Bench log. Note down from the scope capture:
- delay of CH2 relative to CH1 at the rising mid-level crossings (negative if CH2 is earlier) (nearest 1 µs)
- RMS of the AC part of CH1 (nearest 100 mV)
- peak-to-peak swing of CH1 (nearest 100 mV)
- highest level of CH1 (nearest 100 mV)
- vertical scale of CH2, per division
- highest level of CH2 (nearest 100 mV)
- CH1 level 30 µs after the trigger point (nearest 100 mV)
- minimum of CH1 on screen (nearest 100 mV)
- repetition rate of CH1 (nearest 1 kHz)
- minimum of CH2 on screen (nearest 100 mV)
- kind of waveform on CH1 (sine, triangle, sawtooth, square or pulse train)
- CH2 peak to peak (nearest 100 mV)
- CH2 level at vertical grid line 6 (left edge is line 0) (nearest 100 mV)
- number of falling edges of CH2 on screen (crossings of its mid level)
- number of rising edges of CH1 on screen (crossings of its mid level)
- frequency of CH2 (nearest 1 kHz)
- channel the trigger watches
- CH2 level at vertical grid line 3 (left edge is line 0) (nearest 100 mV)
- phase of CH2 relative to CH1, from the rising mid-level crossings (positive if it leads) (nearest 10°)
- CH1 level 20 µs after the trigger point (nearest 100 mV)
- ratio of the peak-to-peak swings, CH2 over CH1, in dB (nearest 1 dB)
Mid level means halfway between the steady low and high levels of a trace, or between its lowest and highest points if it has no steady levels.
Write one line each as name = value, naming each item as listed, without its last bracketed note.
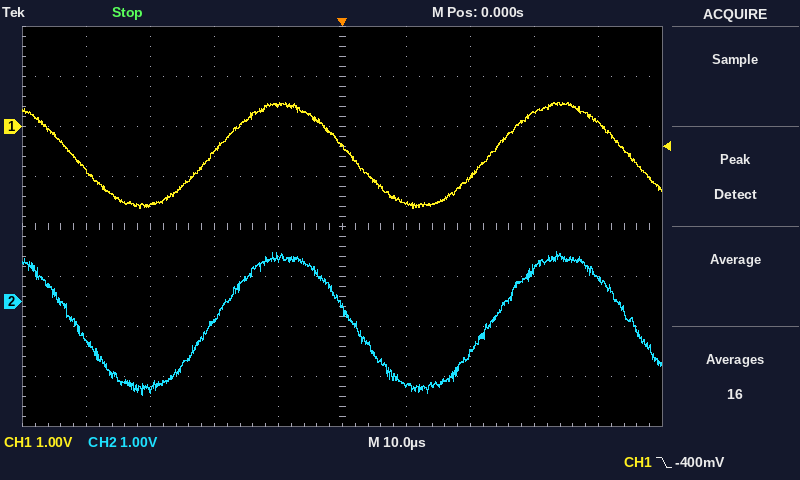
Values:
delay of CH2 relative to CH1 at the rising mid-level crossings (negative if CH2 is earlier) = 0 µs
RMS of the AC part of CH1 = 700 mV
peak-to-peak swing of CH1 = 2.1 V
highest level of CH1 = 500 mV
vertical scale of CH2, per division = 1 V
highest level of CH2 = 1.0 V
CH1 level 30 µs after the trigger point = 300 mV
minimum of CH1 on screen = -1.6 V
repetition rate of CH1 = 23 kHz
minimum of CH2 on screen = -1.9 V
kind of waveform on CH1 = sine
CH2 peak to peak = 2.9 V
CH2 level at vertical grid line 6 (left edge is line 0) = -1.7 V
number of falling edges of CH2 on screen = 3
number of rising edges of CH1 on screen = 2
frequency of CH2 = 23 kHz
channel the trigger watches = CH1
CH2 level at vertical grid line 3 (left edge is line 0) = -400 mV
phase of CH2 relative to CH1, from the rising mid-level crossings (positive if it leads) = 0°
CH1 level 20 µs after the trigger point = -1.0 V
ratio of the peak-to-peak swings, CH2 over CH1, in dB = 3 dB
